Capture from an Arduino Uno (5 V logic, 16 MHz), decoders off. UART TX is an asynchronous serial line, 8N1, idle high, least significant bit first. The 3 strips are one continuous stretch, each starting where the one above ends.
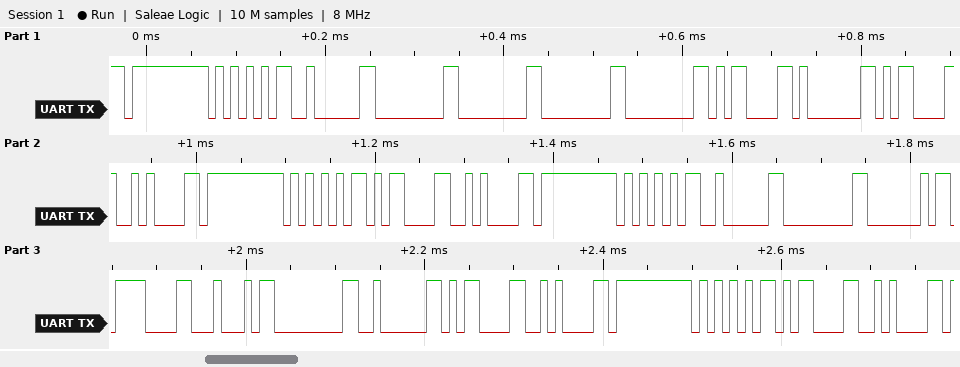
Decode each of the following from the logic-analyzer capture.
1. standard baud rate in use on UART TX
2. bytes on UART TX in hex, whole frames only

115200 baud
FF 55 02 00 00 00 00 0D 01 0D 0A FF 55 0D 0A FF 55 02 00 40 0F 44 00 02 0D 0A FF 55 0D 0A
